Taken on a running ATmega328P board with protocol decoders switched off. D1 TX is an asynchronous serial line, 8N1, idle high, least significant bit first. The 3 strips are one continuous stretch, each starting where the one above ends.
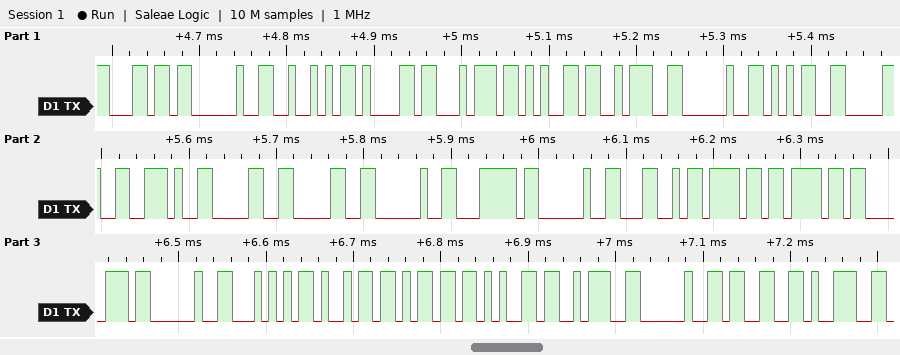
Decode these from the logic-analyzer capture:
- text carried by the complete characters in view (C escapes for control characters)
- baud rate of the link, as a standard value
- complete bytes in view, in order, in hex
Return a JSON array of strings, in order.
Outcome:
["\"l Rate: 50.00 | Loop Time: 39\"", "115200 baud", "6C 20 52 61 74 65 3A 20 35 30 2E 30 30 20 7C 20 4C 6F 6F 70 20 54 69 6D 65 3A 20 33 39"]
